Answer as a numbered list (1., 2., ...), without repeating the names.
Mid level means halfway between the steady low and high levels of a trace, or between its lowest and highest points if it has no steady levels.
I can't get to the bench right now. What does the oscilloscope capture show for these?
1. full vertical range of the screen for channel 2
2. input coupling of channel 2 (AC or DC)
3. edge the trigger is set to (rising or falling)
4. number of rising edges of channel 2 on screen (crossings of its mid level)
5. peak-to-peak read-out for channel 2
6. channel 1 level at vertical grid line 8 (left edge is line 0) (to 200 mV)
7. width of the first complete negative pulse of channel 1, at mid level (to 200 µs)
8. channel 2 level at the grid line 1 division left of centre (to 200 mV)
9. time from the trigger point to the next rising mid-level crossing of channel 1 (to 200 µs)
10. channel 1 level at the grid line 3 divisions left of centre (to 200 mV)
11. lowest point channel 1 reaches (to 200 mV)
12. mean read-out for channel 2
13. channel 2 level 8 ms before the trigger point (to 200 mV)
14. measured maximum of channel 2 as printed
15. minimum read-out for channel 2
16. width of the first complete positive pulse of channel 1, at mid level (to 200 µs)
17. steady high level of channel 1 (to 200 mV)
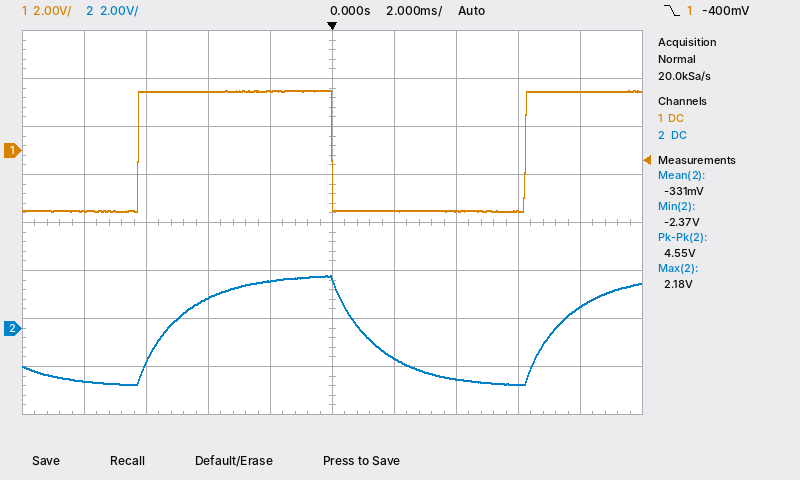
1. 16 V
2. DC
3. falling
4. 2
5. 4.55 V
6. -2.6 V
7. 6.2 ms
8. 2.0 V
9. 6.2 ms
10. 2.4 V
11. -2.6 V
12. -331 mV
13. -2.2 V
14. 2.18 V
15. -2.37 V
16. 6.2 ms
17. 2.4 V
